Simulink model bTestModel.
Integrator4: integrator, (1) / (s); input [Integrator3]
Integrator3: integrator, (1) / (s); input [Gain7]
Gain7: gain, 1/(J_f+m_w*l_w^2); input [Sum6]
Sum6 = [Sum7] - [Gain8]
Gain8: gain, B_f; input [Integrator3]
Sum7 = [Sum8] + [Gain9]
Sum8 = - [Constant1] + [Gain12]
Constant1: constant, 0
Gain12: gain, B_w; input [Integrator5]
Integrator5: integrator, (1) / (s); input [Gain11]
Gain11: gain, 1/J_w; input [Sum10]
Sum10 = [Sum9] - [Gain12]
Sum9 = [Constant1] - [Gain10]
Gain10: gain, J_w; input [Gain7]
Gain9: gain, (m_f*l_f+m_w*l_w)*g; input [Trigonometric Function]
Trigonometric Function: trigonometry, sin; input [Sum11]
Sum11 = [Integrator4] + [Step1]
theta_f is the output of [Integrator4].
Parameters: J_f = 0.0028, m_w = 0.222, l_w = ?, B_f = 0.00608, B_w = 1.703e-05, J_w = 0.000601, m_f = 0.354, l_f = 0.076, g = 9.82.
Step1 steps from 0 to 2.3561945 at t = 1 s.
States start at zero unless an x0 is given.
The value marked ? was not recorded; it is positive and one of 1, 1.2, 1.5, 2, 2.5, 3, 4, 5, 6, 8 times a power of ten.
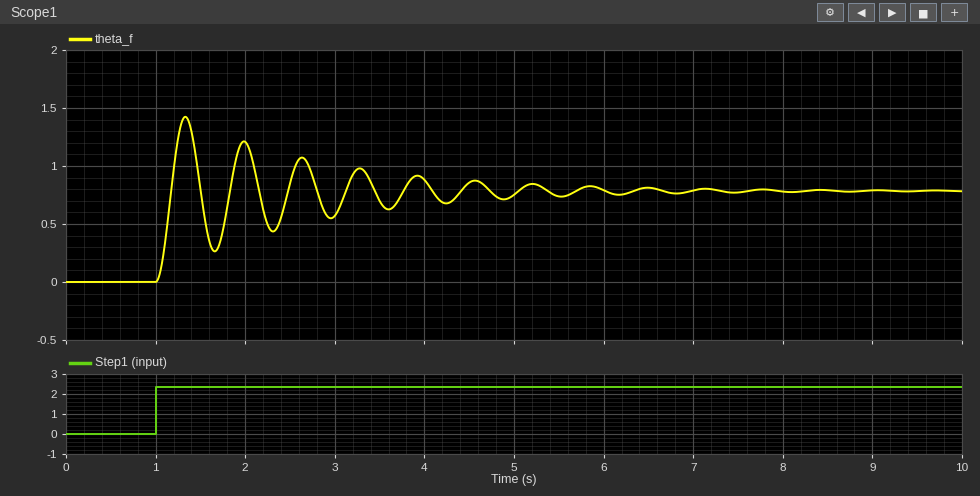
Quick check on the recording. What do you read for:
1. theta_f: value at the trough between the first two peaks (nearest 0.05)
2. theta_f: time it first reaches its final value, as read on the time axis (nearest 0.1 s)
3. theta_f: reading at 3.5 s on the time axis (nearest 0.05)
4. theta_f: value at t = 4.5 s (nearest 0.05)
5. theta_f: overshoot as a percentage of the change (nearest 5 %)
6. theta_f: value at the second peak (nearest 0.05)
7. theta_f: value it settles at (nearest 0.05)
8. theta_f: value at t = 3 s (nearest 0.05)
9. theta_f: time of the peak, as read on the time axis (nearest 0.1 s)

0.25
1.2 s
0.70
0.85
80 %
1.20
0.80
0.55
1.3 s
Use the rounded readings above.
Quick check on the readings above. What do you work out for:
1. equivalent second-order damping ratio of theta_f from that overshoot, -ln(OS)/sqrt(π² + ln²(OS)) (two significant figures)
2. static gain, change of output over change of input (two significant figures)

0.071
0.34
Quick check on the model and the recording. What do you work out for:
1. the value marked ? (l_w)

0.1
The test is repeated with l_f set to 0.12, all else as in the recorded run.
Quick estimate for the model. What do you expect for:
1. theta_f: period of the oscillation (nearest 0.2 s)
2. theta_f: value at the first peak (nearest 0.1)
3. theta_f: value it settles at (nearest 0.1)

0.6 s
1.4
0.8
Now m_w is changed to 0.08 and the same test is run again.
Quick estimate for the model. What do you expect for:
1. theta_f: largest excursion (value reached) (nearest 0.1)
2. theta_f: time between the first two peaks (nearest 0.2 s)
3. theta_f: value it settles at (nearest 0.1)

1.4
0.6 s
0.8
